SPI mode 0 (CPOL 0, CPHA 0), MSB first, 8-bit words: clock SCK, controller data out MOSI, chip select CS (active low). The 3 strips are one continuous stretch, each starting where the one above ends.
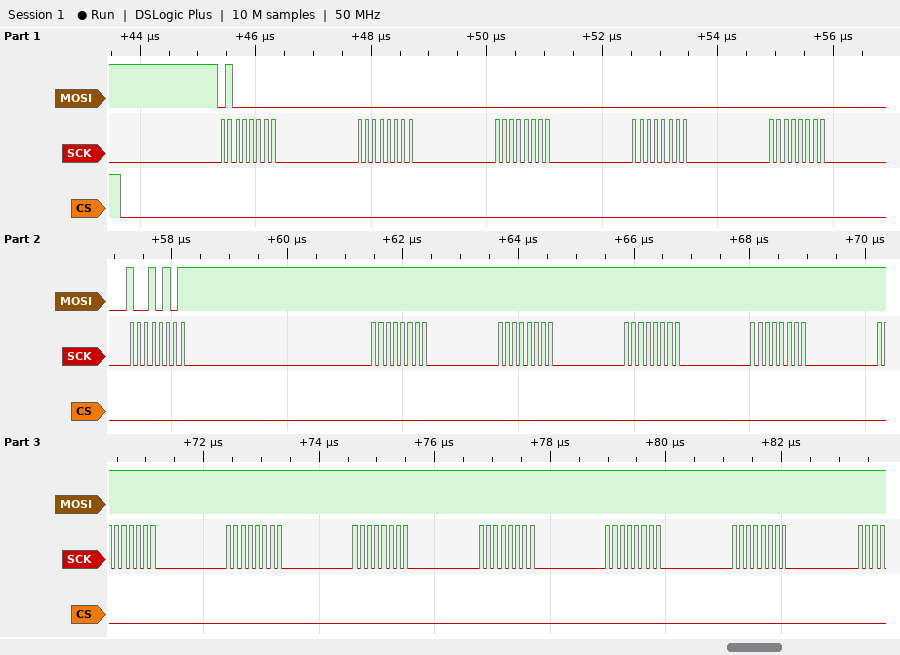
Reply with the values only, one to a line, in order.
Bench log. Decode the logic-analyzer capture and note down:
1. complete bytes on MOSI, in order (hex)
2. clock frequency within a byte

40 00 00 00 00 95 FF FF FF FF FF FF FF FF FF FF
8 MHz
